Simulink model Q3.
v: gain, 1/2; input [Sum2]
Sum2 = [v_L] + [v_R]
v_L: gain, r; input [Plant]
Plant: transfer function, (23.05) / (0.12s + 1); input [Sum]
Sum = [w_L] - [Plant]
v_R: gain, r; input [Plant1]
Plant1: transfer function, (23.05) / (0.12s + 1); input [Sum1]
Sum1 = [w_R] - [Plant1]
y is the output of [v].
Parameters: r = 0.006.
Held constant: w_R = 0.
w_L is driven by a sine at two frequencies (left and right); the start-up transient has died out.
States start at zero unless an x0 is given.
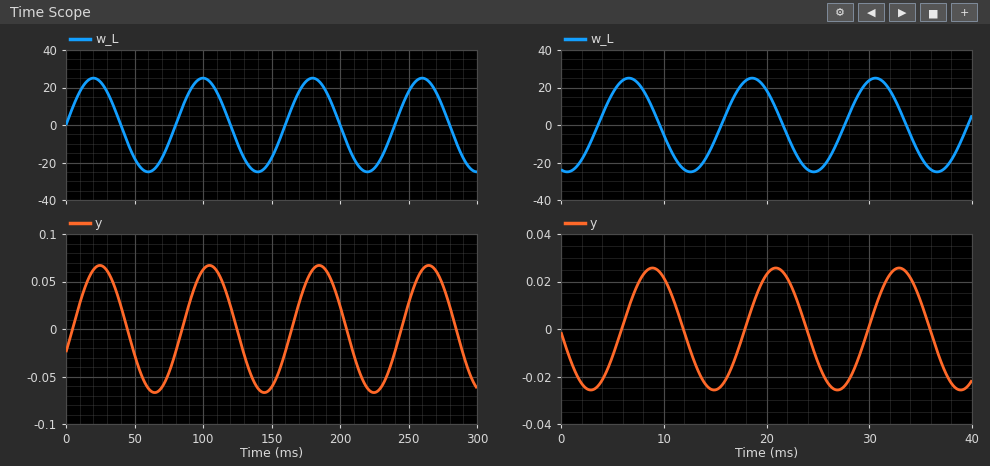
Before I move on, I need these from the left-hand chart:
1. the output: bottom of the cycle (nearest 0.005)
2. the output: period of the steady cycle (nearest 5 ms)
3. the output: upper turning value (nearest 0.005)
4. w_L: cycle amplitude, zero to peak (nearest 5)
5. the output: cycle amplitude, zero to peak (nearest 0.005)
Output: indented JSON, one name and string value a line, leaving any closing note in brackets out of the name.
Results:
{
  "the output: bottom of the cycle": "-0.065",
  "the output: period of the steady cycle": "80 ms",
  "the output: upper turning value": "0.065",
  "w_L: cycle amplitude, zero to peak": "25",
  "the output: cycle amplitude, zero to peak": "0.065"
}
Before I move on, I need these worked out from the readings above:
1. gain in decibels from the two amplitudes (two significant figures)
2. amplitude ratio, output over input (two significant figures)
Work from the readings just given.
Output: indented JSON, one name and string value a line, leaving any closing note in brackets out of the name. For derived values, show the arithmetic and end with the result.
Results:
{
  "gain in decibels from the two amplitudes": "20 log10(0.065 / 25) = -52 dB",
  "amplitude ratio, output over input": "0.065 / 25 = 0.0026"
}
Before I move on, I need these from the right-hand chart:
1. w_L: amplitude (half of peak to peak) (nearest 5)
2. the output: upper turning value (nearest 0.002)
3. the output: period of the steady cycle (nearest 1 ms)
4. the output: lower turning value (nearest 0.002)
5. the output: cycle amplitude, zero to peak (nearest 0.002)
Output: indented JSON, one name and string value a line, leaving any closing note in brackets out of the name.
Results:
{
  "w_L: amplitude (half of peak to peak)": "25",
  "the output: upper turning value": "0.026",
  "the output: period of the steady cycle": "12 ms",
  "the output: lower turning value": "-0.026",
  "the output: cycle amplitude, zero to peak": "0.026"
}
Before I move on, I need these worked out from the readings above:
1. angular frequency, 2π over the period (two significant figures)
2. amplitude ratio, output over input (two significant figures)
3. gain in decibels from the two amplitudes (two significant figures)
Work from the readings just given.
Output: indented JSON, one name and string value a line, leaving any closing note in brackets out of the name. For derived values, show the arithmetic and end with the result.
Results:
{
  "angular frequency, 2π over the period": "2π / 12 = 0.52 rad/ms",
  "amplitude ratio, output over input": "0.026 / 25 = 0.0010",
  "gain in decibels from the two amplitudes": "20 log10(0.026 / 25) = -60 dB"
}
